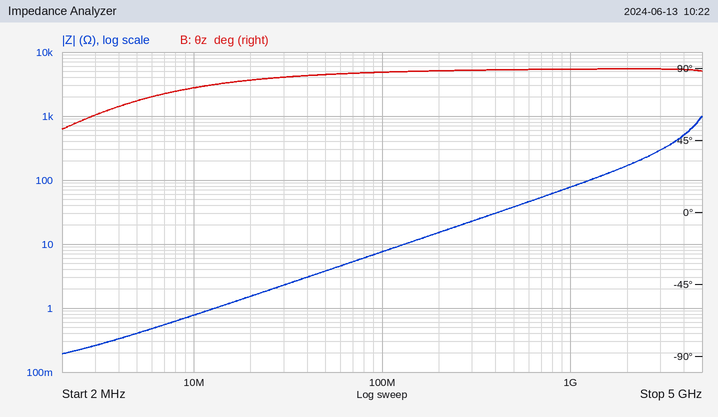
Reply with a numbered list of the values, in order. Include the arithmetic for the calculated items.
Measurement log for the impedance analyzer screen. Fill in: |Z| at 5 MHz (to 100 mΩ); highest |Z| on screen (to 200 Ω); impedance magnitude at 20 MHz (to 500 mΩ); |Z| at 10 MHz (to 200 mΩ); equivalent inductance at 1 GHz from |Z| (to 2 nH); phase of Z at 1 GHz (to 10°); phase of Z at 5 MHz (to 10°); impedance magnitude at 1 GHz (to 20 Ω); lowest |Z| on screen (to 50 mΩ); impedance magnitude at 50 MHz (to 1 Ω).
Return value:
1. 400 mΩ
2. 1.0 kΩ
3. 1.5 Ω
4. 800 mΩ
5. L = 80 Ω/(2π × 1 GHz) ≈ 12.7 nH, so 12 nH to the nearest 2 nH
6. 90°
7. 70°
8. 80 Ω
9. 200 mΩ
10. 4 Ω
